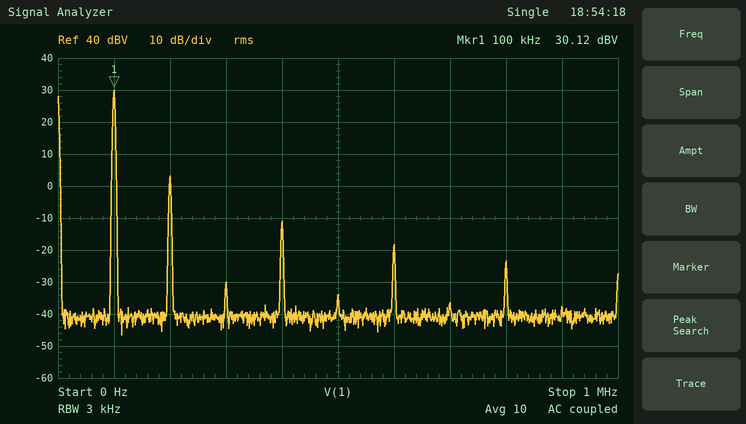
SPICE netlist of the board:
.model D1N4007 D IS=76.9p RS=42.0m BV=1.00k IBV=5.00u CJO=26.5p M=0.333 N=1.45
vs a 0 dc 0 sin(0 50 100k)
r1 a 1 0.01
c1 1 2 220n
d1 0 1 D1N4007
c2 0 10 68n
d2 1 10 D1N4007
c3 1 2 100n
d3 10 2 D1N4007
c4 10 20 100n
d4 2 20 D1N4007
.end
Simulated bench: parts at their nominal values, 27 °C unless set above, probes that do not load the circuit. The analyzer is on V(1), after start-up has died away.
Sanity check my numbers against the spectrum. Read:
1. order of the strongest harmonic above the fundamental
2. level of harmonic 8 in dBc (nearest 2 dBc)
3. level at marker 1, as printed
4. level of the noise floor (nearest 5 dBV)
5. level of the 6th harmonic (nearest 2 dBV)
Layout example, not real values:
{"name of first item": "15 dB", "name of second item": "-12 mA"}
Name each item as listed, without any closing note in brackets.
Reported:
{"order of the strongest harmonic above the fundamental": "2", "level of harmonic 8 in dBc": "-54 dBc", "level at marker 1, as printed": "30.12 dBV", "level of the noise floor": "-40 dBV", "level of the 6th harmonic": "-18 dBV"}
